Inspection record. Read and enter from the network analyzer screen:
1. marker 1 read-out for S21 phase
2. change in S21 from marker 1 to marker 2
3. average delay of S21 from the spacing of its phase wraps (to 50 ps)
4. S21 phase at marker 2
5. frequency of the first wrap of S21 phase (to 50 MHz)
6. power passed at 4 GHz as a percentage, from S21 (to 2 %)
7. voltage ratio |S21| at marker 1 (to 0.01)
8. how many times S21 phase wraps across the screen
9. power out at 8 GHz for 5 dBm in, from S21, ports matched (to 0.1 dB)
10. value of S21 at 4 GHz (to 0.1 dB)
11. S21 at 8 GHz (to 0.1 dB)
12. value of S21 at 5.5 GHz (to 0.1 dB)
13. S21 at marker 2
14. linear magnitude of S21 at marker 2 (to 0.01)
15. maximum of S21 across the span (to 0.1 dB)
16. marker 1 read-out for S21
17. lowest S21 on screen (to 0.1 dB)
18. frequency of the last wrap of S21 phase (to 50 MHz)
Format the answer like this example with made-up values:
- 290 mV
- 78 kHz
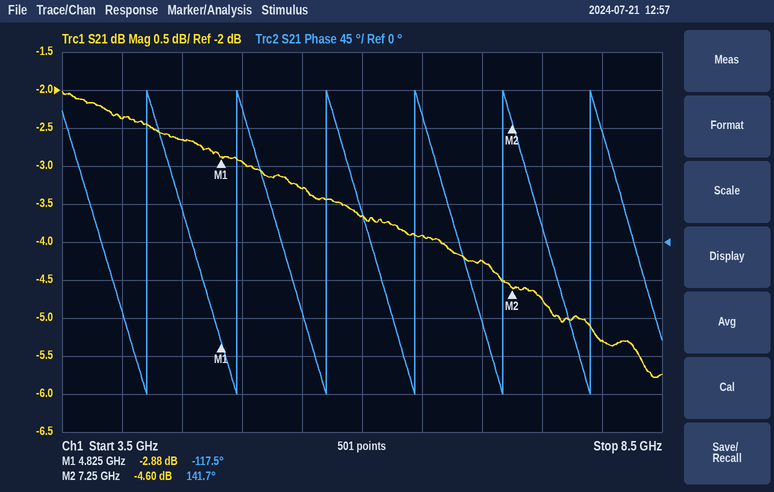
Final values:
- -117.5°
- -1.72 dB
- 1.35 ns
- 141.7°
- 4.20 GHz
- 58 %
- 0.72
- 6
- -0.3 dBm
- -2.4 dB
- -5.3 dB
- -3.3 dB
- -4.60 dB
- 0.59
- -2.0 dB
- -2.88 dB
- -5.8 dB
- 7.90 GHz
